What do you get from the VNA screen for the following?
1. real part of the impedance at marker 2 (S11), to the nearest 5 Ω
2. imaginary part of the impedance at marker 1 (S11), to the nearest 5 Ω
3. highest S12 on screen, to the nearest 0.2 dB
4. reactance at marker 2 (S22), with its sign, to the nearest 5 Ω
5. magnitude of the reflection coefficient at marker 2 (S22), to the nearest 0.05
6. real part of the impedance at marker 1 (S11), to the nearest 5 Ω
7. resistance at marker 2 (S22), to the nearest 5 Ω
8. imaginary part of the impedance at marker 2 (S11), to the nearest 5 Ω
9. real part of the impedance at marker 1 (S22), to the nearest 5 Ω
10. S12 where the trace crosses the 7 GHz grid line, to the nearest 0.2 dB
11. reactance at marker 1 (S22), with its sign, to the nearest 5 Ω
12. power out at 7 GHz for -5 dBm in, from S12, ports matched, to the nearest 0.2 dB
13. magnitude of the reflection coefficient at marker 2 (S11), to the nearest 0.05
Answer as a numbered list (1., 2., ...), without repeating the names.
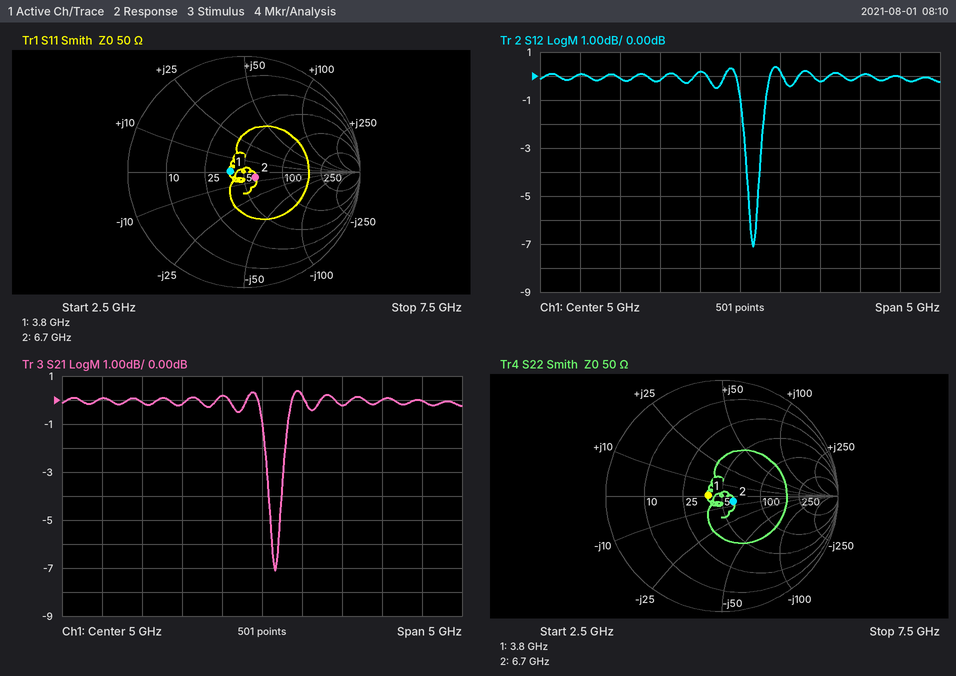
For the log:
1. 60 Ω
2. 0 Ω
3. 0.4 dB
4. -5 Ω
5. 0.10
6. 40 Ω
7. 60 Ω
8. -5 Ω
9. 40 Ω
10. 0.0 dB
11. 0 Ω
12. -5.0 dBm
13. 0.10
